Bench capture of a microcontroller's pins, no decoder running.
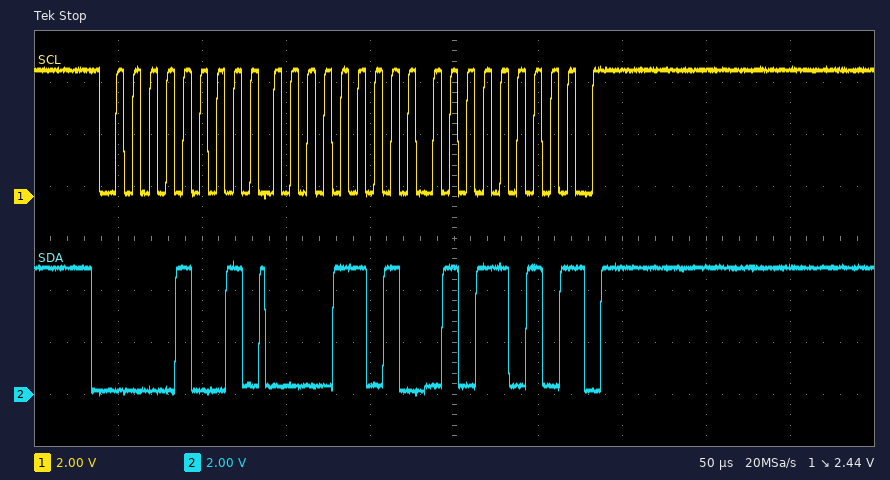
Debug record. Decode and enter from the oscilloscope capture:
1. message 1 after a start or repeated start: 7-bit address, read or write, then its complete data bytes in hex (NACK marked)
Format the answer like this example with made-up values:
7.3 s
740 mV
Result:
0x04 read: 0D 5A NACK
